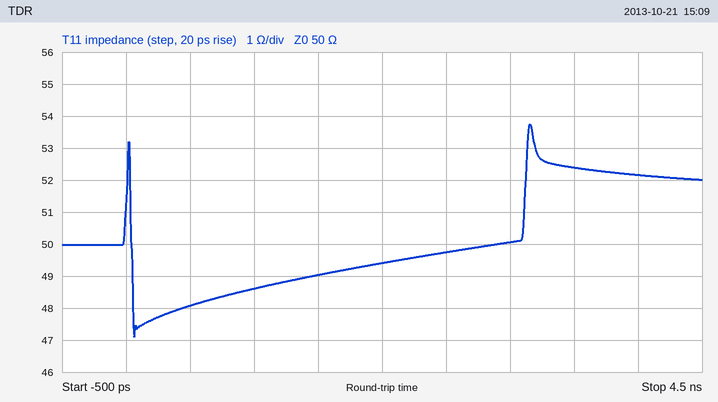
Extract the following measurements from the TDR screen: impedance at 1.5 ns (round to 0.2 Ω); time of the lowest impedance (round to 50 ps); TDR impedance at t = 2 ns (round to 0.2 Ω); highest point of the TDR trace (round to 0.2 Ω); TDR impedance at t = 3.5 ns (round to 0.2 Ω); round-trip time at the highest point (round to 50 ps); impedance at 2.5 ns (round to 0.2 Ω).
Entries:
49.0 Ω
50 ps
49.4 Ω
53.8 Ω
52.4 Ω
3.15 ns
49.8 Ω
